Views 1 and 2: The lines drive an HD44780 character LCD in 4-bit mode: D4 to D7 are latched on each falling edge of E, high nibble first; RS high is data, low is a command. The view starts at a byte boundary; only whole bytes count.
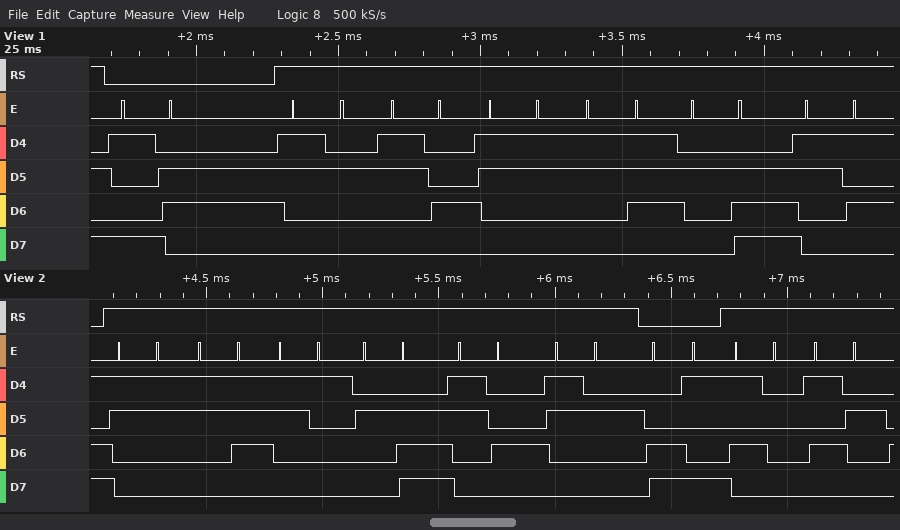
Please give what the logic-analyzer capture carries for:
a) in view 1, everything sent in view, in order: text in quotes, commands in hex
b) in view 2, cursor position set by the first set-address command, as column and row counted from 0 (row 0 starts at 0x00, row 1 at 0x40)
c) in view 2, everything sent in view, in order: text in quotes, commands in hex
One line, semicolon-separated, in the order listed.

0x96 "2437.5"; column 9, row 1; "371.42" 0xC9 "PR"
